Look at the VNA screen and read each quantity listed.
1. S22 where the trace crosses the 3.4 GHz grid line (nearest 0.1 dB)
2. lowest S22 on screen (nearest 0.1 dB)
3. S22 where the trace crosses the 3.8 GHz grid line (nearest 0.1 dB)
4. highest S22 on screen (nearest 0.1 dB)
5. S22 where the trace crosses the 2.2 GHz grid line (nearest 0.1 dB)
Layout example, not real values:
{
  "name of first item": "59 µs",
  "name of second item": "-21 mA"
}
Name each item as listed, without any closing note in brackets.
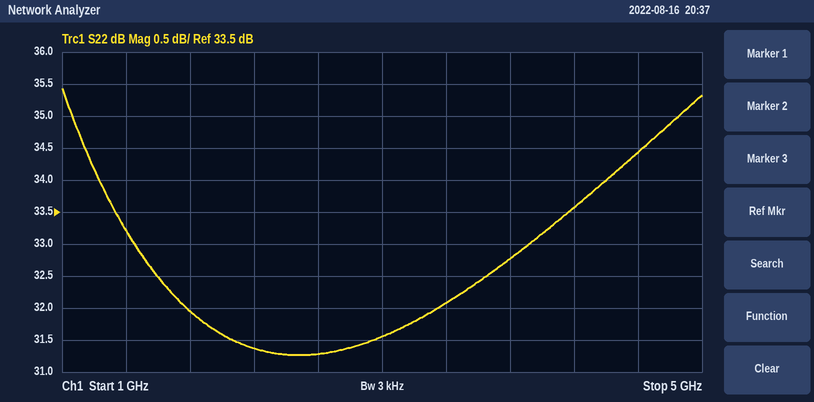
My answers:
{
  "S22 where the trace crosses the 3.4 GHz grid line": "32.1 dB",
  "lowest S22 on screen": "31.3 dB",
  "S22 where the trace crosses the 3.8 GHz grid line": "32.8 dB",
  "highest S22 on screen": "35.4 dB",
  "S22 where the trace crosses the 2.2 GHz grid line": "31.4 dB"
}
